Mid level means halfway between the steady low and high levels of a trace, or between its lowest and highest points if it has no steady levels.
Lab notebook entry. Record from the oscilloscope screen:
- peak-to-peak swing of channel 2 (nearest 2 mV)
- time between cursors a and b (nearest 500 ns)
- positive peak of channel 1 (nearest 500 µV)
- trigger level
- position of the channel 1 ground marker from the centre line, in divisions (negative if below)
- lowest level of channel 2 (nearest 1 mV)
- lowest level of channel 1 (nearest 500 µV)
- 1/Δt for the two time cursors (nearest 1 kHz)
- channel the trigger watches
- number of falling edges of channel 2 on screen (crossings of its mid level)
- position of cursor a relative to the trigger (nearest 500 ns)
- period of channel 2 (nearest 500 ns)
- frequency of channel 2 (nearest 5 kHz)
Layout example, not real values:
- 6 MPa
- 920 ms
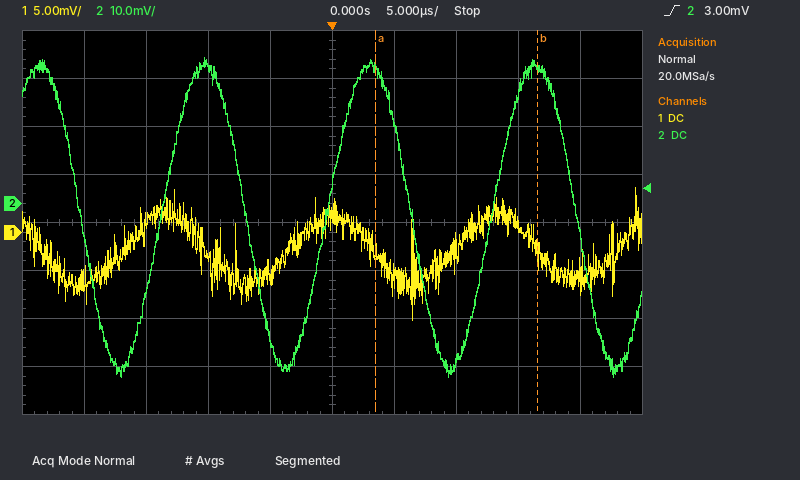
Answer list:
- 66 mV
- 13.0 µs
- 4.5 mV
- 3.00 mV
- -0.2 div
- -36 mV
- -9.0 mV
- 77 kHz
- channel 2
- 4
- +3.5 µs
- 13.5 µs
- 75 kHz
